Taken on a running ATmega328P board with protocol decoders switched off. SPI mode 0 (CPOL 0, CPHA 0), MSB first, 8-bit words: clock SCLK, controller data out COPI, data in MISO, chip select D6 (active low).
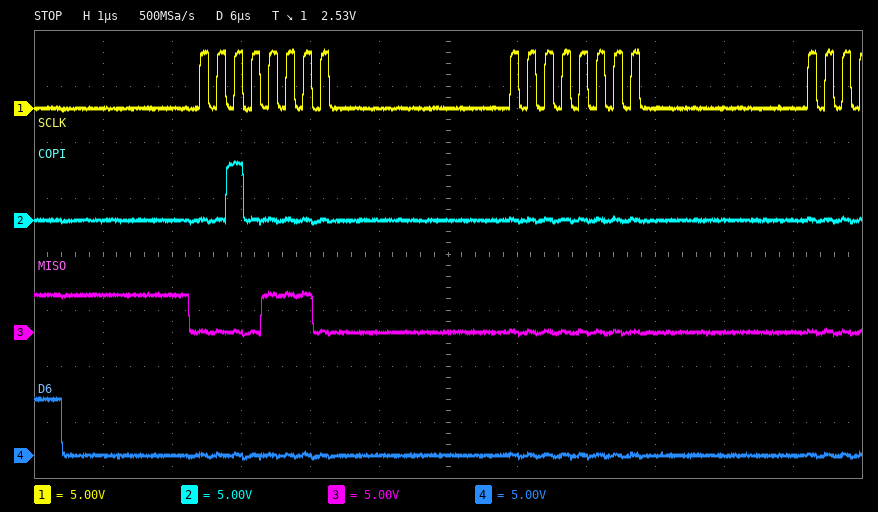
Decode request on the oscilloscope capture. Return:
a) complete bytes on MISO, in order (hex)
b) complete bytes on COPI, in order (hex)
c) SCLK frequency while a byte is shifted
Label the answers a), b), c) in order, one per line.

a) 0E 00
b) 20 00
c) 4 MHz
